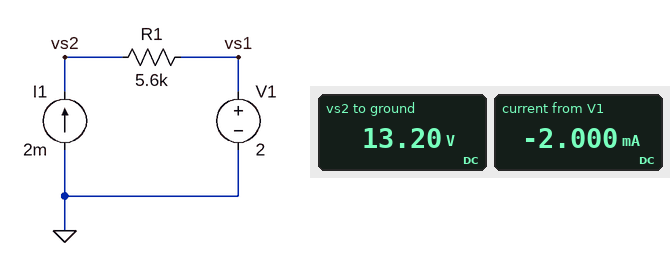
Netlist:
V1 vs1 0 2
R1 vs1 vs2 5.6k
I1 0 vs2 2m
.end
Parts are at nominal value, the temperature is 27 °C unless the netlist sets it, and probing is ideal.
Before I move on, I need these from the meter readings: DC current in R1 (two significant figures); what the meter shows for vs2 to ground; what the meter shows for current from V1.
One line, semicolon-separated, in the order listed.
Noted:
2.0 mA; 13.20 V; -2.000 mA
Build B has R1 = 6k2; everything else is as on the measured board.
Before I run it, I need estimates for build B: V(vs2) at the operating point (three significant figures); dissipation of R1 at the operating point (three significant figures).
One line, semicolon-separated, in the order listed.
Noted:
14.4 V; 24.8 mW
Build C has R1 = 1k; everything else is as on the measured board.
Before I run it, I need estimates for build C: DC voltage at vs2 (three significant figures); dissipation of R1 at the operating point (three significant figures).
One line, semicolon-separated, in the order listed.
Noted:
4.00 V; 4.00 mW
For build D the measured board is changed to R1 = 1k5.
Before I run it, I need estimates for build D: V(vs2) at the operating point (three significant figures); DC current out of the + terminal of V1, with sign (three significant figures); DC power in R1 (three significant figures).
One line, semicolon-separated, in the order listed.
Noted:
5.00 V; -2.00 mA; 6.00 mW
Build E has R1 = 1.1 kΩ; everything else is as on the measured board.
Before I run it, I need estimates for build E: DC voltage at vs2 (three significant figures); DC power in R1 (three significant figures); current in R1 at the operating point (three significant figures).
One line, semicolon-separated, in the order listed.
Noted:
4.20 V; 4.40 mW; 2.00 mA
